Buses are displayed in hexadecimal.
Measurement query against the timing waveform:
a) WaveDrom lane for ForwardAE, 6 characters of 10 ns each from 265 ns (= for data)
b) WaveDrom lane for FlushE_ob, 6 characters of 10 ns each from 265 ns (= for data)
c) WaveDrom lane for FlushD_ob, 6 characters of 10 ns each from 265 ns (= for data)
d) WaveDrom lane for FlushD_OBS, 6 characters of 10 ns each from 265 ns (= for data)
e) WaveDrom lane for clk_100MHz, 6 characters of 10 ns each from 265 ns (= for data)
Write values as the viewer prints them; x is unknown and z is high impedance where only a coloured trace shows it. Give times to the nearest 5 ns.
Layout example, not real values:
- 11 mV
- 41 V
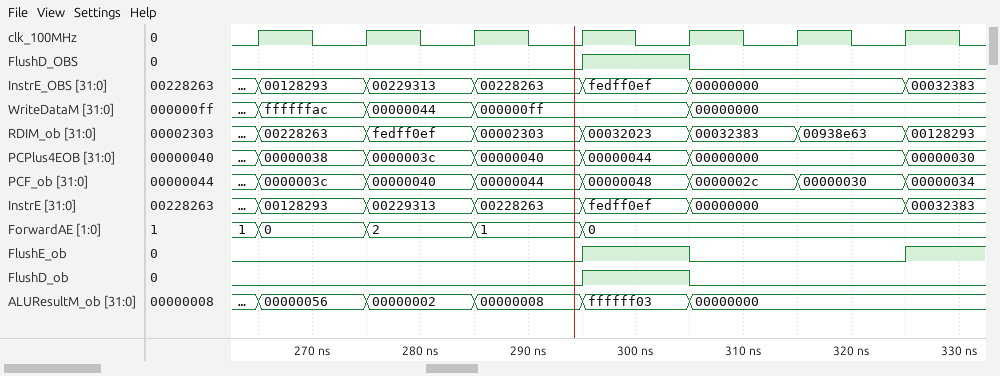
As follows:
- {name: 'ForwardAE', wave: '====..', data: '0 2 1 0'}
- {name: 'FlushE_ob', wave: '0..10.'}
- {name: 'FlushD_ob', wave: '0..10.'}
- {name: 'FlushD_OBS', wave: '0..10.'}
- {name: 'clk_100MHz', wave: 'p.....'}
